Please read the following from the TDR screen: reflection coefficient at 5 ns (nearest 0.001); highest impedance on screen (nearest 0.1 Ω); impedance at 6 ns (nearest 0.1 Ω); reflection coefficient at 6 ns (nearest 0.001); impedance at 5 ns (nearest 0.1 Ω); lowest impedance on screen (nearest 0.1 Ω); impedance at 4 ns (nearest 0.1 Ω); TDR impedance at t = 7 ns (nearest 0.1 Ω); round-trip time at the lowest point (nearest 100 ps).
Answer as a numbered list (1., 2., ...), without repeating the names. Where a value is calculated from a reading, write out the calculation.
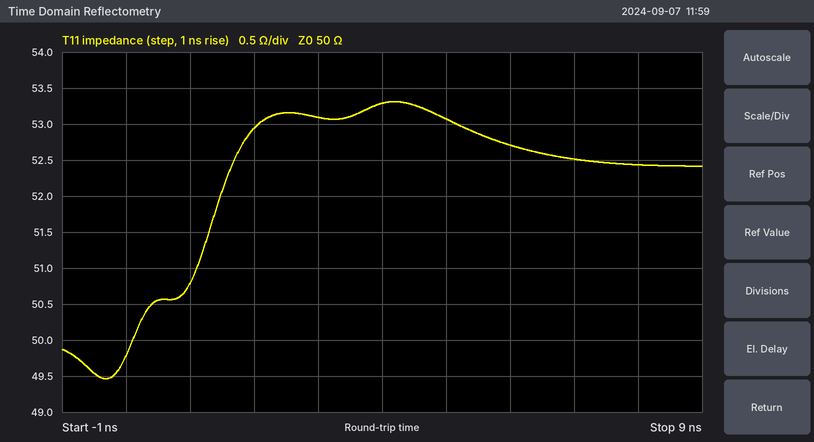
1. (53.1 − 50)/(53.1 + 50) ≈ +0.030
2. 53.3 Ω
3. 52.7 Ω
4. (52.7 − 50)/(52.7 + 50) ≈ +0.026
5. 53.1 Ω
6. 49.5 Ω
7. 53.3 Ω
8. 52.5 Ω
9. -300 ps
